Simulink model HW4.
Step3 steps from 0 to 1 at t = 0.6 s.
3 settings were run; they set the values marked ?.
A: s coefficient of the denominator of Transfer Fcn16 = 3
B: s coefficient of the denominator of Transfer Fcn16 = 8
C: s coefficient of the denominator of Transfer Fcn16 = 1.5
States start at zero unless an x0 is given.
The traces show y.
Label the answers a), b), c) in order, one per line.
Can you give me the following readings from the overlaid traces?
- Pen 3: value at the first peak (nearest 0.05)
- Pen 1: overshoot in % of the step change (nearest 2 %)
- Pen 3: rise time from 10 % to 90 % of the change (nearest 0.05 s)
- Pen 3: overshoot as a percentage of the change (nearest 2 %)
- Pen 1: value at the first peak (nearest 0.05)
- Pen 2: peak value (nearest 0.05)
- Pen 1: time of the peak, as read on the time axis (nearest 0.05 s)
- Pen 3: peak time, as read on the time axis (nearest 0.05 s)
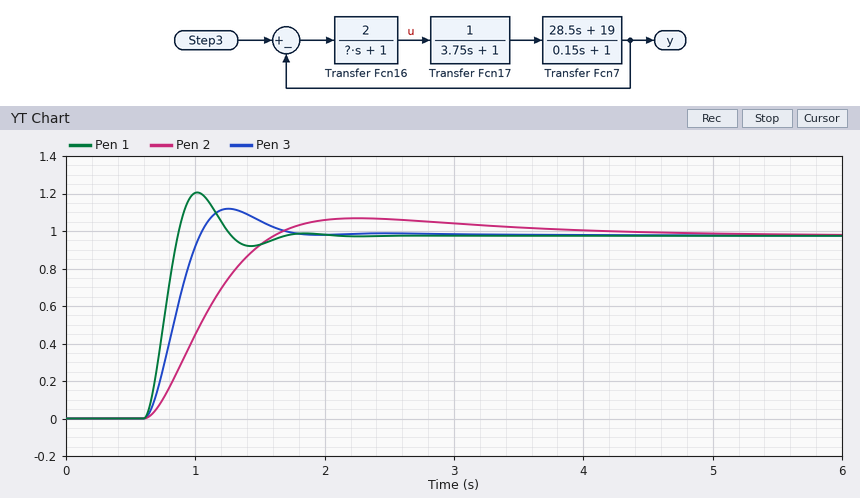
a) 1.10
b) 24 %
c) 0.30 s
d) 14 %
e) 1.20
f) 1.05
g) 1.00 s
h) 1.25 s
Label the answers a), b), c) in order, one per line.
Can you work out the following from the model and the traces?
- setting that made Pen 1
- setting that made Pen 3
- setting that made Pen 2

a) C
b) A
c) B
